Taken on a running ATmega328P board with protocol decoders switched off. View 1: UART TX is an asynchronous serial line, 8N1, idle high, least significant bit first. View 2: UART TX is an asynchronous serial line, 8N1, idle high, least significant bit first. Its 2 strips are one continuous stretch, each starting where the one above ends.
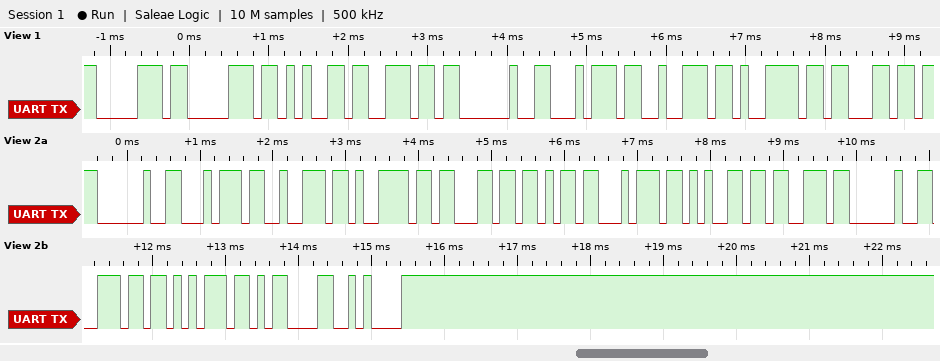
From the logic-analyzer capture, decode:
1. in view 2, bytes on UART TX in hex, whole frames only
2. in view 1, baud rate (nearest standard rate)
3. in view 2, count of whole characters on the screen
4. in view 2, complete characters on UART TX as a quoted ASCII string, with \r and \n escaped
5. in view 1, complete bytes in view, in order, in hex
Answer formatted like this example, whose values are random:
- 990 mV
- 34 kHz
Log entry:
- 20 74 72 79 63 6B 74 65 73 20 6E 75 0D 0A
- 9600 baud
- 14
- " trycktes nu\r\n"
- 70 70 65 6E 20 74 72 79 63
